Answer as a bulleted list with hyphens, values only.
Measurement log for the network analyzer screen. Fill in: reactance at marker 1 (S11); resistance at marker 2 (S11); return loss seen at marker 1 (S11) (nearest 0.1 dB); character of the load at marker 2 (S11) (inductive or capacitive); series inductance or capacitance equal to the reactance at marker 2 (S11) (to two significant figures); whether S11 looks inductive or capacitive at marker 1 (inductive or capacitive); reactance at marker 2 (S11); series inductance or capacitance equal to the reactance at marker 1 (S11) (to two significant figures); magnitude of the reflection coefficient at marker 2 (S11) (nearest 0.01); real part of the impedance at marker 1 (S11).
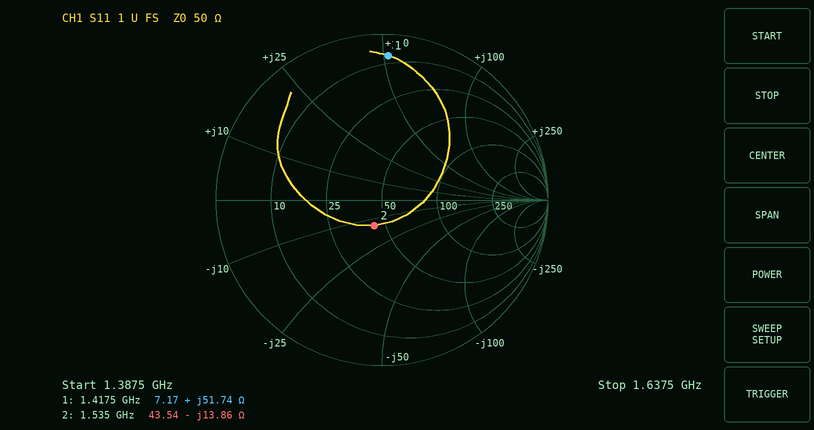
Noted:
- +51.74 Ω
- 43.54 Ω
- 1.2 dB
- capacitive
- 7.5 pF
- inductive
- -13.86 Ω
- 5.8 nH
- 0.16
- 7.17 Ω
